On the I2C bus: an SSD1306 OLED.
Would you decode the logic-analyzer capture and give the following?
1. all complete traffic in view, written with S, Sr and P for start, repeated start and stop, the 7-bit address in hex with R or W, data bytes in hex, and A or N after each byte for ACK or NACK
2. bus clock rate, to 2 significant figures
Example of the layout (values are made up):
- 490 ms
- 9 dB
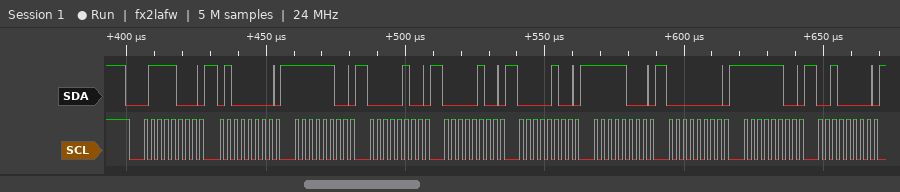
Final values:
- S 3CW A 40 A FC A 04 A 04 A 04 A F8 A 00 A FC A 20 A
- 400 kHz
